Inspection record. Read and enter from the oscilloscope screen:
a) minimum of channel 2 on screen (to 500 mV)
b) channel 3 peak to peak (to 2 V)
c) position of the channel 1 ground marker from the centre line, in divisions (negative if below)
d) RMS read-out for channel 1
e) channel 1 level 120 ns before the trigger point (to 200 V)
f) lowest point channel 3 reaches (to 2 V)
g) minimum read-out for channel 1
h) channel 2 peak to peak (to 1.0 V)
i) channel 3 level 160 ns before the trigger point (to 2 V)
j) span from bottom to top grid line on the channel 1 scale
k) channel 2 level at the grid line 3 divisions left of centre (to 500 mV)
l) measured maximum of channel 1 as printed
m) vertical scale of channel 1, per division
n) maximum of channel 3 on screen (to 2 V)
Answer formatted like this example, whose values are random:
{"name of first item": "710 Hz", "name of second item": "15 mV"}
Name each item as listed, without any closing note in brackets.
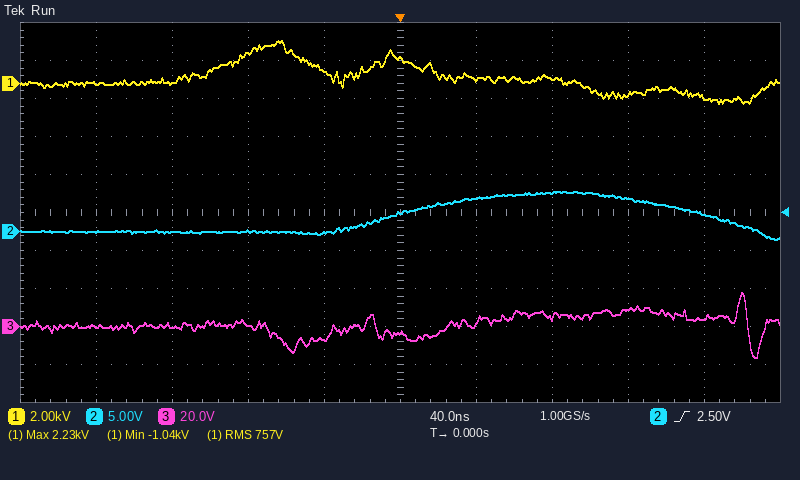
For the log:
{"minimum of channel 2 on screen": "-1.0 V", "channel 3 peak to peak": "34 V", "position of the channel 1 ground marker from the centre line, in divisions": "+3.4 div", "RMS read-out for channel 1": "757 V", "channel 1 level 120 ns before the trigger point": "0.0 kV", "lowest point channel 3 reaches": "-16 V", "minimum read-out for channel 1": "-1.04 kV", "channel 2 peak to peak": "6.0 V", "channel 3 level 160 ns before the trigger point": "0 V", "span from bottom to top grid line on the channel 1 scale": "20 kV", "channel 2 level at the grid line 3 divisions left of centre": "0.0 V", "measured maximum of channel 1 as printed": "2.23 kV", "vertical scale of channel 1, per division": "2 kV", "maximum of channel 3 on screen": "18 V"}
